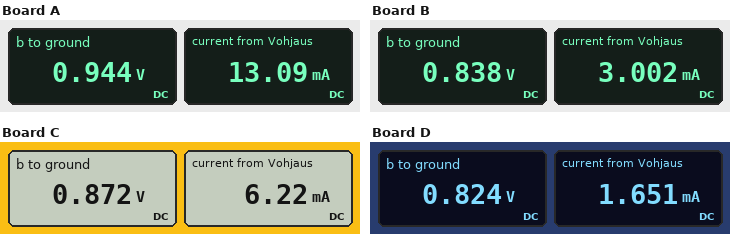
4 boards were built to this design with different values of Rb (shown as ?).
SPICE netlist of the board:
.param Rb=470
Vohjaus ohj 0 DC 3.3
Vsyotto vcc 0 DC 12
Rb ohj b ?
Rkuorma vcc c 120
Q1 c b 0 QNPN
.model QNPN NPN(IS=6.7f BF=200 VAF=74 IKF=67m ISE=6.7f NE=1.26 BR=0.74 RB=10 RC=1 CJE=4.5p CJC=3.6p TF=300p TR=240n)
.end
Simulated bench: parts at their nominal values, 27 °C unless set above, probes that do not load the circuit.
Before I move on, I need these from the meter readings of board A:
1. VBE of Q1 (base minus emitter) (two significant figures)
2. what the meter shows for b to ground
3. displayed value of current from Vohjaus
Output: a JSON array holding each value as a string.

["940 mV", "0.944 V", "13.09 mA"]
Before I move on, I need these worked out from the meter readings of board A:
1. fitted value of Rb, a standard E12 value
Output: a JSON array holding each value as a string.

["180 Ω"]
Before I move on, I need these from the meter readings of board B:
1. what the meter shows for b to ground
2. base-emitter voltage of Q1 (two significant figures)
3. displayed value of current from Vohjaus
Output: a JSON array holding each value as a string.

["0.838 V", "840 mV", "3.002 mA"]
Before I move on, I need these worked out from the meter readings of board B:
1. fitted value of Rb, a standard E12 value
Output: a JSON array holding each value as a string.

["820 Ω"]
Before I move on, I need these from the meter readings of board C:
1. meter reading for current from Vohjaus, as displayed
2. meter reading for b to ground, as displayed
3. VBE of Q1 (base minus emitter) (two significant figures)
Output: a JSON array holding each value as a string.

["6.22 mA", "0.872 V", "870 mV"]
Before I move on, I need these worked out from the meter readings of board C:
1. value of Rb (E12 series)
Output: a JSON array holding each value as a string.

["390 Ω"]
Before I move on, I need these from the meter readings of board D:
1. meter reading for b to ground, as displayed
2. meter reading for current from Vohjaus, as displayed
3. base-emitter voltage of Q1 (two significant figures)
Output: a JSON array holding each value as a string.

["0.824 V", "1.651 mA", "820 mV"]
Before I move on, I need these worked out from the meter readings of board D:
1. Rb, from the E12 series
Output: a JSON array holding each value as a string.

["1.5 kΩ"]
